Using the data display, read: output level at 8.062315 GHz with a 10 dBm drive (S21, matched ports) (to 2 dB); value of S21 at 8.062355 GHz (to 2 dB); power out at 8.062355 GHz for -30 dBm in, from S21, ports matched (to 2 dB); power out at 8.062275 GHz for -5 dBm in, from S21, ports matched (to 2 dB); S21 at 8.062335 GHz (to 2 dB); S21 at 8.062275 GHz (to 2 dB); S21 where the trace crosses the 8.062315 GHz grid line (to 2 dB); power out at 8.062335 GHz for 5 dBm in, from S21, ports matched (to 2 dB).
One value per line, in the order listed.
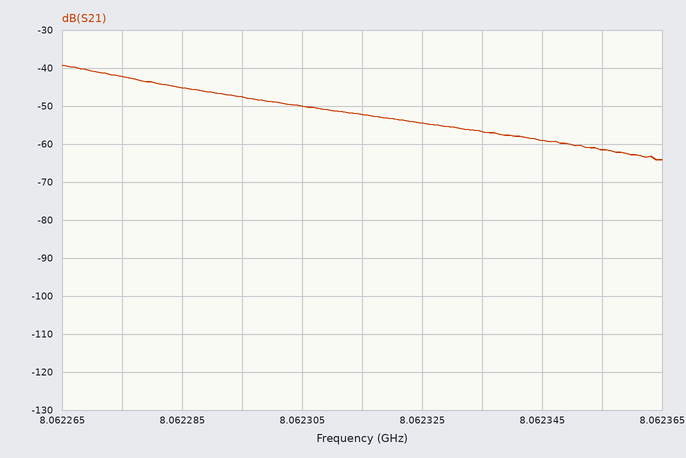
-42 dBm
-62 dB
-92 dBm
-48 dBm
-56 dB
-42 dB
-52 dB
-52 dBm
